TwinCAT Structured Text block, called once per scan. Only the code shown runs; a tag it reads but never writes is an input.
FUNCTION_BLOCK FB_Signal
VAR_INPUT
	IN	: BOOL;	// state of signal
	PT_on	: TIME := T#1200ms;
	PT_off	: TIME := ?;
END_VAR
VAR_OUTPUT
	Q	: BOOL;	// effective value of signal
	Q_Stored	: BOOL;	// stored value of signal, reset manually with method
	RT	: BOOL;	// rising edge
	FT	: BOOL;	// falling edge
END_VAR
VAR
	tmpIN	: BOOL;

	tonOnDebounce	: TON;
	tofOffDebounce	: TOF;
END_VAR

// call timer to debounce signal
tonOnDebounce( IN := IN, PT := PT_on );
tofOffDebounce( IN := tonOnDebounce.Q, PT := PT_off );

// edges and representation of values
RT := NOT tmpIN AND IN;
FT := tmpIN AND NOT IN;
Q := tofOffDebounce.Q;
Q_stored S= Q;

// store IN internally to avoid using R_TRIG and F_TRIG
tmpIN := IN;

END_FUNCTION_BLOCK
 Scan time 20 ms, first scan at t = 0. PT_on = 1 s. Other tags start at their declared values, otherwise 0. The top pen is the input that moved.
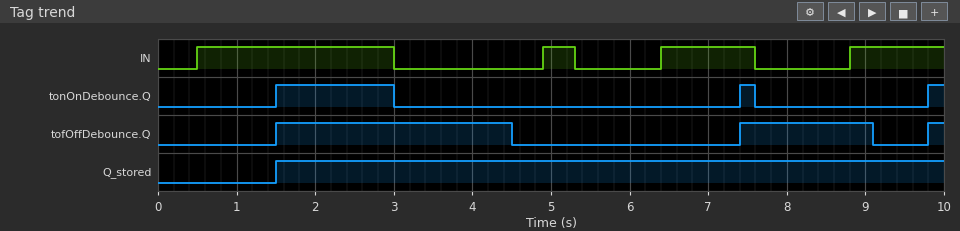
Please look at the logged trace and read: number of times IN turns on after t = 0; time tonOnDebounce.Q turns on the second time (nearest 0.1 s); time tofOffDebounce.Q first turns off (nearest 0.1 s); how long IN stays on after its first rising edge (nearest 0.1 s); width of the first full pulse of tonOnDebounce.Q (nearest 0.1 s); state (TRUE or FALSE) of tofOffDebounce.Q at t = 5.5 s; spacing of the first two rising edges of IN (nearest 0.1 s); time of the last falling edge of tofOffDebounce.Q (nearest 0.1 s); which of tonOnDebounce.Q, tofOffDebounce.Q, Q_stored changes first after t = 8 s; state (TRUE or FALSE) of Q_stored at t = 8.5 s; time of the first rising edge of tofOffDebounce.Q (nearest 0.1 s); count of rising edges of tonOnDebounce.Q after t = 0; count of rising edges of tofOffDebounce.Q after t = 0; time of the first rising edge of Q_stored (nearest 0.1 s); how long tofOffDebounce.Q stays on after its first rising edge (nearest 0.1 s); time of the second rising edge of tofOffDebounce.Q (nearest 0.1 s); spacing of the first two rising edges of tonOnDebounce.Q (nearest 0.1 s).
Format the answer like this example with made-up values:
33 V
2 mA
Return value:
4
7.4 s
4.5 s
2.5 s
1.5 s
FALSE
4.4 s
9.1 s
tofOffDebounce.Q
TRUE
1.5 s
3
3
1.5 s
3.0 s
7.4 s
5.9 s
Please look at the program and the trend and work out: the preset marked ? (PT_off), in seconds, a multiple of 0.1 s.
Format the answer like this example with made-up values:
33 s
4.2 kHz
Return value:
1.5 s
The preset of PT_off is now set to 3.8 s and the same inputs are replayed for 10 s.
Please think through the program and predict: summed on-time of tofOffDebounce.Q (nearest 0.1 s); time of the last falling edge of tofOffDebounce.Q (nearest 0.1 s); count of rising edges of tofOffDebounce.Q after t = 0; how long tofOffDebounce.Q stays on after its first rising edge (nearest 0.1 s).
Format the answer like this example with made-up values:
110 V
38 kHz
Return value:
7.9 s
6.8 s
2
5.3 s
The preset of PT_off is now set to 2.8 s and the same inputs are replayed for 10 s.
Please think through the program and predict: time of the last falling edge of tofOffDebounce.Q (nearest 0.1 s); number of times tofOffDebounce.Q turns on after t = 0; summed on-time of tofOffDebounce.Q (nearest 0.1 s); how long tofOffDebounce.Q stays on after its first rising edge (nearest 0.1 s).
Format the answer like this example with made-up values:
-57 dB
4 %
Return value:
5.8 s
2
6.9 s
4.3 s
